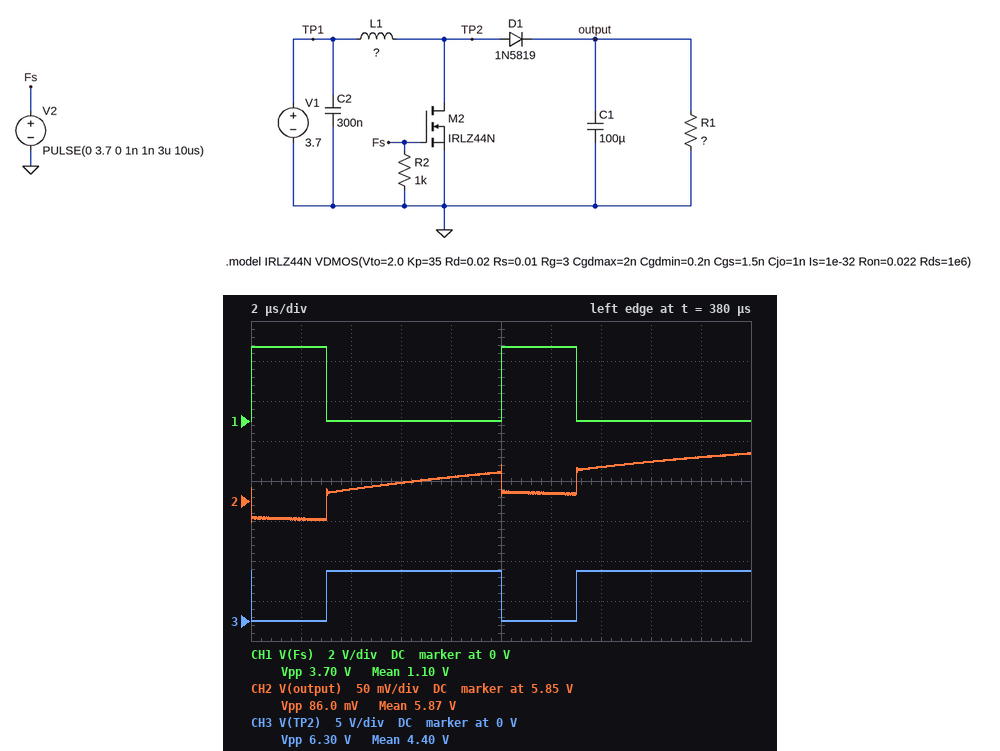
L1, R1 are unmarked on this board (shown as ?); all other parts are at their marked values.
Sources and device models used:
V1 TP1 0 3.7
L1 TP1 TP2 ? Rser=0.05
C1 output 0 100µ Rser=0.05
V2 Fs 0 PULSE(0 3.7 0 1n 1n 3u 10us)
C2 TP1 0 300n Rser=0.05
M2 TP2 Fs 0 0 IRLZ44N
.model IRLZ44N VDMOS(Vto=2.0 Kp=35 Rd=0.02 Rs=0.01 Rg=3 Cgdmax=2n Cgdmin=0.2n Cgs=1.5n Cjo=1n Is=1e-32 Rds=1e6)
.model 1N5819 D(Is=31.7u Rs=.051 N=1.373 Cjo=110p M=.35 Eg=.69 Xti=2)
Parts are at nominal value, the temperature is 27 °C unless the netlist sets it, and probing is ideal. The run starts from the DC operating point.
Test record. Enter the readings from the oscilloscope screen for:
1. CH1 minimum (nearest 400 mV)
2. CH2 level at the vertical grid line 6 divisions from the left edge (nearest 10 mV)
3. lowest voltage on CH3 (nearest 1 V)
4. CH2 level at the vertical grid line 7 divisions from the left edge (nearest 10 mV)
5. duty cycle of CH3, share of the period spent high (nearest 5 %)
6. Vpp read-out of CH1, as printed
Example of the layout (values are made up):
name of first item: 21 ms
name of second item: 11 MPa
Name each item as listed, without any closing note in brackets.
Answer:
CH1 minimum: 0 V
CH2 level at the vertical grid line 6 divisions from the left edge: 5.86 V
lowest voltage on CH3: 0 V
CH2 level at the vertical grid line 7 divisions from the left edge: 5.89 V
duty cycle of CH3, share of the period spent high: 70 %
Vpp read-out of CH1, as printed: 3.70 V
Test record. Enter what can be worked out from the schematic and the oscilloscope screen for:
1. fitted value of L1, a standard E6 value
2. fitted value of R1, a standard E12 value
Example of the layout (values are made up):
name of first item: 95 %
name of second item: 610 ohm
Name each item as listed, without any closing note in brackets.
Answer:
fitted value of L1, a standard E6 value: 100 µH
fitted value of R1, a standard E12 value: 68 Ω
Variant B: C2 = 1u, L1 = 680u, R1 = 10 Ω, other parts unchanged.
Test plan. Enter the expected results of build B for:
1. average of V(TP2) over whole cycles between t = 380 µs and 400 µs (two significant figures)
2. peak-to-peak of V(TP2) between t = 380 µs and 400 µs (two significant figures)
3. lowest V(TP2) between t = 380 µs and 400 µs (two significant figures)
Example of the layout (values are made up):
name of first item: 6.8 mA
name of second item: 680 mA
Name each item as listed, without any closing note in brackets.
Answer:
average of V(TP2) over whole cycles between t = 380 µs and 400 µs: 2.9 V
peak-to-peak of V(TP2) between t = 380 µs and 400 µs: 4.2 V
lowest V(TP2) between t = 380 µs and 400 µs: 20 mV
